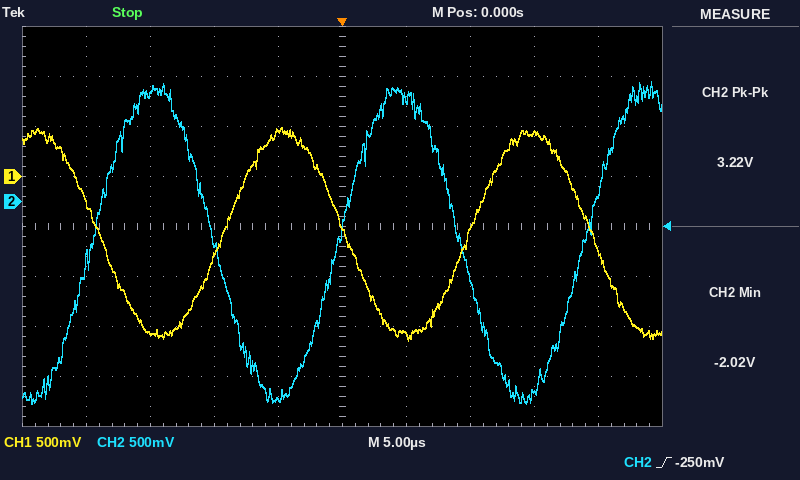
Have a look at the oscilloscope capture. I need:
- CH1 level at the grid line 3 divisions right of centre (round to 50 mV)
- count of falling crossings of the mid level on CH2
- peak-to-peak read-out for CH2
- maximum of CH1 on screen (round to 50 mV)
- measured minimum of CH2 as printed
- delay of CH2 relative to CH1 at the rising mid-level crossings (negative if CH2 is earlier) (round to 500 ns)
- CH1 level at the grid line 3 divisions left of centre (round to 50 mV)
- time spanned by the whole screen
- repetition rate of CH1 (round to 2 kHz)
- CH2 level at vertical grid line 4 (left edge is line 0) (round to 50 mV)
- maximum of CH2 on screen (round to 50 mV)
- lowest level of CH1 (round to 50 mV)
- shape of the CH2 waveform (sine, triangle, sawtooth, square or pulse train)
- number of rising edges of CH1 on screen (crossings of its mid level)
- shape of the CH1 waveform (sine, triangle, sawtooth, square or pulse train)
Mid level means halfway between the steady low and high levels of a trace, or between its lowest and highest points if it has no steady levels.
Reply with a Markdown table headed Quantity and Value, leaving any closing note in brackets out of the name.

| Quantity | Value |
|---|---|
| CH1 level at the grid line 3 divisions right of centre | 450 mV |
| count of falling crossings of the mid level on CH2 | 2 |
| peak-to-peak read-out for CH2 | 3.22 V |
| maximum of CH1 on screen | 500 mV |
| measured minimum of CH2 as printed | -2.02 V |
| delay of CH2 relative to CH1 at the rising mid-level crossings (negative if CH2 is earlier) | +9.0 µs |
| CH1 level at the grid line 3 divisions left of centre | -1.55 V |
| time spanned by the whole screen | 50 µs |
| repetition rate of CH1 | 52 kHz |
| CH2 level at vertical grid line 4 (left edge is line 0) | -2.00 V |
| maximum of CH2 on screen | 1.20 V |
| lowest level of CH1 | -1.65 V |
| shape of the CH2 waveform | sine |
| number of rising edges of CH1 on screen | 2 |
| shape of the CH1 waveform | sine |
